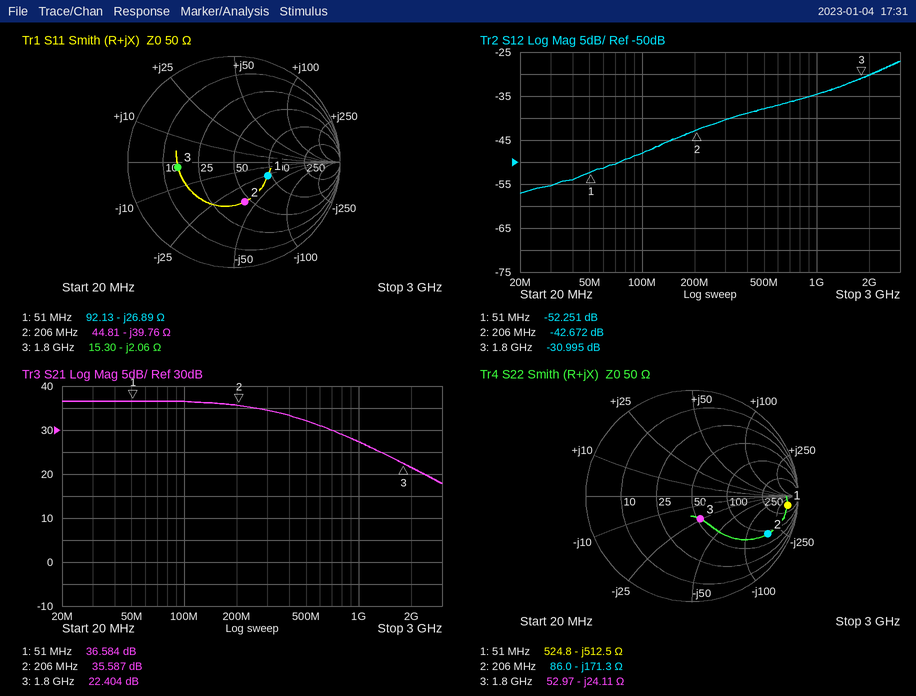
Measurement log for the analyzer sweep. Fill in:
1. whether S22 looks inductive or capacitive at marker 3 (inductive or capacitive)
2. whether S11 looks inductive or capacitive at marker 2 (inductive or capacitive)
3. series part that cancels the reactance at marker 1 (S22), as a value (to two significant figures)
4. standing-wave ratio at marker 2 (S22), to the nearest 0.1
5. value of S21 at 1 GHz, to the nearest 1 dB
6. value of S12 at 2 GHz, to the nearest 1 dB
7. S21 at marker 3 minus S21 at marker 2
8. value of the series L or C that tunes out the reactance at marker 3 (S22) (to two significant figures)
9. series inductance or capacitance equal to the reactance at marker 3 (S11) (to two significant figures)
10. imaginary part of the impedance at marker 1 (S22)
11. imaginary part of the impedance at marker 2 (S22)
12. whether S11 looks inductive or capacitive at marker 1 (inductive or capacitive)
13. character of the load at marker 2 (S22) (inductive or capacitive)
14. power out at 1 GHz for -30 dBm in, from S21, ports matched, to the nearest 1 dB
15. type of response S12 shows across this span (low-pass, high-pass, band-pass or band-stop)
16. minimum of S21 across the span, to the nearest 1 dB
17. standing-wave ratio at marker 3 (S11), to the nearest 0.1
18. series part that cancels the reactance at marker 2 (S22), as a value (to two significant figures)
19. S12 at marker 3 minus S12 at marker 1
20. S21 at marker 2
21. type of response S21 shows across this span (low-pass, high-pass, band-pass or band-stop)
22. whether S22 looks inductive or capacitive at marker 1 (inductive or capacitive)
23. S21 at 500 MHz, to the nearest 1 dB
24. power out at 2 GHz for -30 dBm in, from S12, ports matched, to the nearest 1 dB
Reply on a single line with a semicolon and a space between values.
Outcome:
capacitive; capacitive; 1.6 µH; 9.0; 27 dB; -30 dB; -13.183 dB; 2.1 nH; 43 pF; -512.5 Ω; -171.3 Ω; capacitive; capacitive; -3 dBm; high-pass; 18 dB; 3.3; 130 nH; 21.256 dB; 35.587 dB; low-pass; capacitive; 32 dB; -60 dBm
